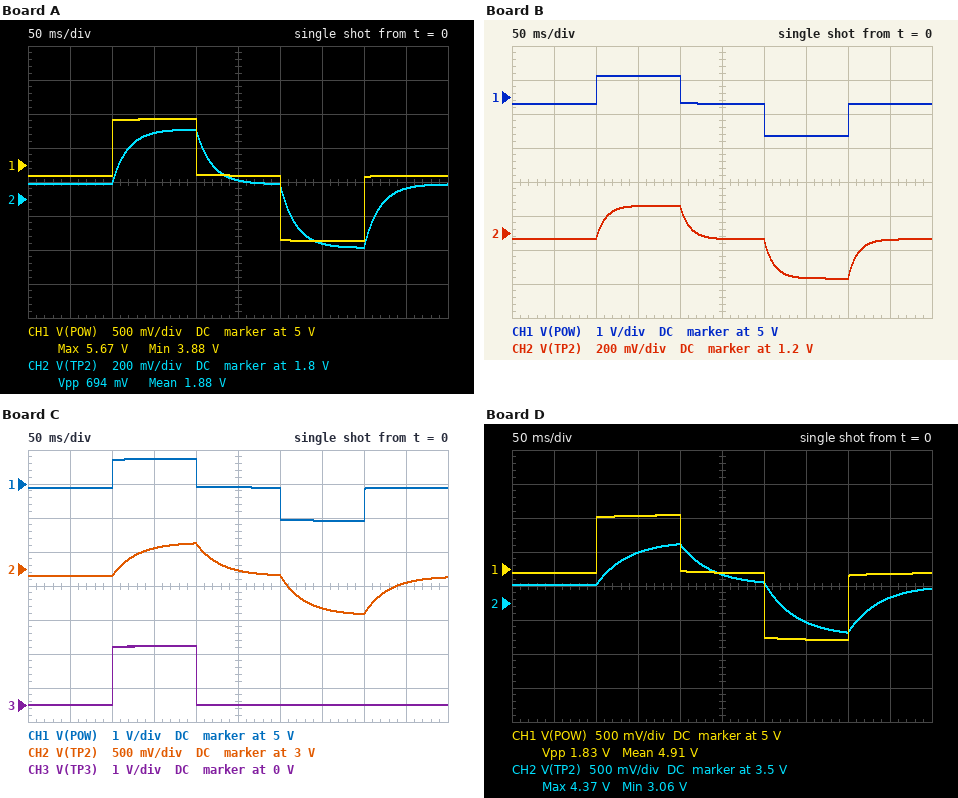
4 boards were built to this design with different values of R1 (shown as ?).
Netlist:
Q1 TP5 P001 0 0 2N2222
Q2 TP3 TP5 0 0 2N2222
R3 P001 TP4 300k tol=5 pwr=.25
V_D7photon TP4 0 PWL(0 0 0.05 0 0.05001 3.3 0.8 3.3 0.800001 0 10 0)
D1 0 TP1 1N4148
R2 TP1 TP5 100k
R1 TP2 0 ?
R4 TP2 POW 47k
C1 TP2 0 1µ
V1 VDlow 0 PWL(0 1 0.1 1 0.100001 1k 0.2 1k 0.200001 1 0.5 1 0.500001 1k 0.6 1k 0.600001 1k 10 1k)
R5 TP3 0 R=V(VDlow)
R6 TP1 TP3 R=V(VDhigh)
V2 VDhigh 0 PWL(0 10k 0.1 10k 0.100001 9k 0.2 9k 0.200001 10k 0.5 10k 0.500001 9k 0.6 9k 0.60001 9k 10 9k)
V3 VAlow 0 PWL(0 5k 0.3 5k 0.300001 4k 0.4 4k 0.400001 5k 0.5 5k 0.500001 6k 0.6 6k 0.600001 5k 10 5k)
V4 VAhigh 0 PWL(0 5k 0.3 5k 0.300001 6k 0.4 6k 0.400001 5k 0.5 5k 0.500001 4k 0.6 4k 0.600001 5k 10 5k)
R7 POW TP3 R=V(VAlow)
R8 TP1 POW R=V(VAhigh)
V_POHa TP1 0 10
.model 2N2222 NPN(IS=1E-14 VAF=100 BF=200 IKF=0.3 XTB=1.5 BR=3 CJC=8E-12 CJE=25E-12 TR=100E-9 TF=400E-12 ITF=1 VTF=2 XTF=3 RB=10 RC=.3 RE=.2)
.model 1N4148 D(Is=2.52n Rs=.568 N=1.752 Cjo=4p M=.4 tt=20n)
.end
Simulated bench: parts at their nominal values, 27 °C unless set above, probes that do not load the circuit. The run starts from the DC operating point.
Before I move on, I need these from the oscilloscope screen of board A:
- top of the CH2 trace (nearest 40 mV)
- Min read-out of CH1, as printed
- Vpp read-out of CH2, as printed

2.20 V
3.88 V
694 mV
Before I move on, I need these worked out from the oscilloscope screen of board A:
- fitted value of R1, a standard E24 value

30 kΩ
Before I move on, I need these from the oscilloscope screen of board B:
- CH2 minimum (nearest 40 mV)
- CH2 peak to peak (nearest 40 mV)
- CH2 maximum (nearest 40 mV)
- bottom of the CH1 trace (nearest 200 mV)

920 mV
440 mV
1.36 V
3.8 V
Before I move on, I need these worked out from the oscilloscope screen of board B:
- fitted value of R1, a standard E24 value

15 kΩ
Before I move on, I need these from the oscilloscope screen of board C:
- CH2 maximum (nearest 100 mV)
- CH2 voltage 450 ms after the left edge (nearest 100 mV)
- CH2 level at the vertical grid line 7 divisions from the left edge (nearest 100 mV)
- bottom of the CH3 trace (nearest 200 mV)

3.4 V
2.8 V
2.4 V
0 V
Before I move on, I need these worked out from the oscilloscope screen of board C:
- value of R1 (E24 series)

68 kΩ
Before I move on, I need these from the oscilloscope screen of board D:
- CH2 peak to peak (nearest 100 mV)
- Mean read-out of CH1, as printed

1.3 V
4.91 V
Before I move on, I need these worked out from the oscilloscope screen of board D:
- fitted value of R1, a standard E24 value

150 kΩ
